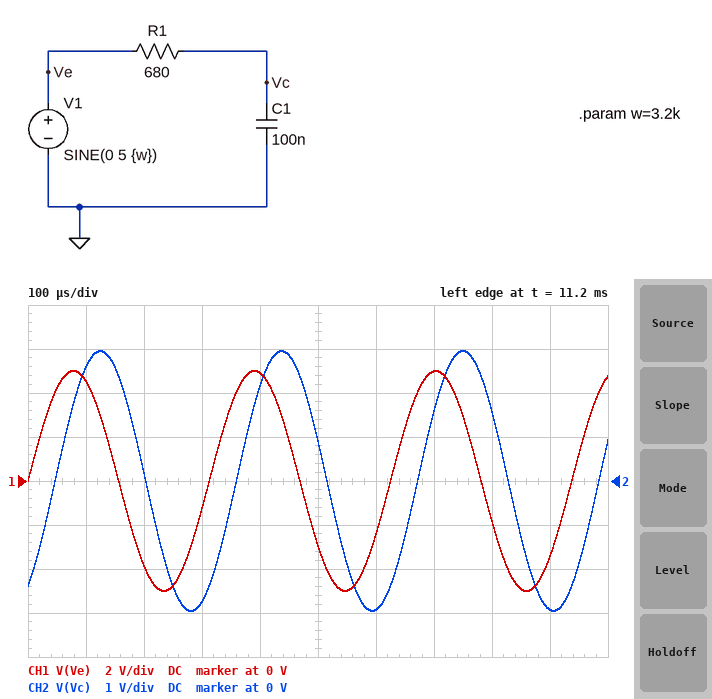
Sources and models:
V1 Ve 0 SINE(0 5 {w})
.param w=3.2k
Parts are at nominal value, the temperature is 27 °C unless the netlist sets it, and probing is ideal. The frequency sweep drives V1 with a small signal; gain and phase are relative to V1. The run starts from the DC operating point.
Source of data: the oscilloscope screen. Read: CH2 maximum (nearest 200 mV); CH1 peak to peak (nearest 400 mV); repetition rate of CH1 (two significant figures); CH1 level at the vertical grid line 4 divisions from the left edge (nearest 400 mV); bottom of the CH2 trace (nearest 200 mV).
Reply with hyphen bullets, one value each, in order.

- 3.0 V
- 10.0 V
- 3.2 kHz
- 4.8 V
- -3.0 V
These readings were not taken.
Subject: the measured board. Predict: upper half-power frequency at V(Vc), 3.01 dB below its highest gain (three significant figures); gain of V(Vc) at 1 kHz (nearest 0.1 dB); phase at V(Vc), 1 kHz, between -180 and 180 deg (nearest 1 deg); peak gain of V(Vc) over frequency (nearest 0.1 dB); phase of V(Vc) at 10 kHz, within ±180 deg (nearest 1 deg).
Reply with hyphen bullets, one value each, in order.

- 2.34 kHz
- -0.7 dB
- -23 deg
- 0 dB
- -77 deg
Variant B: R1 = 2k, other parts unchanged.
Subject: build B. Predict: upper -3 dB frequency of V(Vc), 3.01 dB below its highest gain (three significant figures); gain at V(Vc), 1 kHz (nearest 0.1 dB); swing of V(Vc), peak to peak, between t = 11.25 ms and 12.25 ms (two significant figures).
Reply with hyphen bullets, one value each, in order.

- 796 Hz
- -4.1 dB
- 2.4 V
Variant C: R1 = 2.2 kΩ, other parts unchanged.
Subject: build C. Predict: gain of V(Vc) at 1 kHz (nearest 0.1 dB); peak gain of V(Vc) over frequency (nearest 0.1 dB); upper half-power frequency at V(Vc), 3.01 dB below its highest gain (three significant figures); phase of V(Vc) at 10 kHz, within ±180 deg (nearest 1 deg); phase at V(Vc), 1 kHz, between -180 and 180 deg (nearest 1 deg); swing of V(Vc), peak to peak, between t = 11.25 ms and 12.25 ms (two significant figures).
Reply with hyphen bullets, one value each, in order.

- -4.6 dB
- 0 dB
- 723 Hz
- -86 deg
- -54 deg
- 2.2 V
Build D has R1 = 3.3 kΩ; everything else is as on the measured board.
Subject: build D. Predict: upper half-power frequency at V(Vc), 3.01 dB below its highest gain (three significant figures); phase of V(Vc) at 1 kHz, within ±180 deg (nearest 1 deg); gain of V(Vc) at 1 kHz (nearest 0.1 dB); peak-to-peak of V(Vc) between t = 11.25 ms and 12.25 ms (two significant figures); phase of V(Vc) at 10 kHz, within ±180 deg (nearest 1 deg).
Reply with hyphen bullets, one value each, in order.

- 482 Hz
- -64 deg
- -7.2 dB
- 1.5 V
- -87 deg
